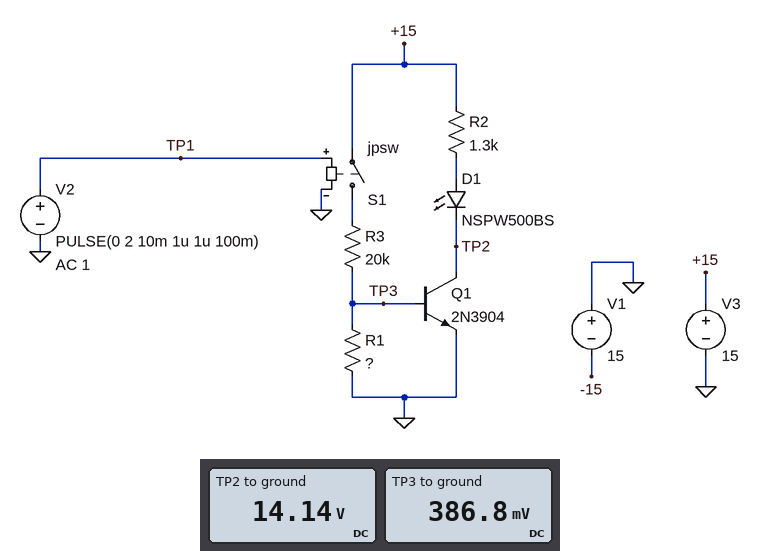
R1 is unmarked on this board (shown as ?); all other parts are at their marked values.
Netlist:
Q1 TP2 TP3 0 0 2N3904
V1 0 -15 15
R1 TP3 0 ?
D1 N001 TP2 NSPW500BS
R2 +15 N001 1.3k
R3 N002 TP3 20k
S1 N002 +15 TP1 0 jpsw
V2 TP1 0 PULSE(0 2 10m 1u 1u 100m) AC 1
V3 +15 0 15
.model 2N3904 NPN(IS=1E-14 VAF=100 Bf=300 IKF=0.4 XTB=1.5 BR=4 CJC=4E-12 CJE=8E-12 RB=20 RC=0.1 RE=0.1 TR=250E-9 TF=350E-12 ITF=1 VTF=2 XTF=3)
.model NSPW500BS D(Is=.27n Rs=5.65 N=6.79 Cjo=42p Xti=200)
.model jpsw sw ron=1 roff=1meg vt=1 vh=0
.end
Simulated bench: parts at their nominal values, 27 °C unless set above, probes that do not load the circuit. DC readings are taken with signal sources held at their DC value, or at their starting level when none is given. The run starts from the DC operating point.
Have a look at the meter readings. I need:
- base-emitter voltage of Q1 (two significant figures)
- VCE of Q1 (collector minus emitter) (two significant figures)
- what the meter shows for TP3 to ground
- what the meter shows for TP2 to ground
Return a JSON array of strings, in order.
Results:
["390 mV", "14 V", "386.8 mV", "14.14 V"]
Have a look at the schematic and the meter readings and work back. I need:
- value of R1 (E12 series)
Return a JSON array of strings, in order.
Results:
["27 kΩ"]
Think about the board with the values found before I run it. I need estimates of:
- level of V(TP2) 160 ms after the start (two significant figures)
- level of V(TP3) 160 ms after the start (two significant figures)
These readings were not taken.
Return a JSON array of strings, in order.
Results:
["14 V", "390 mV"]
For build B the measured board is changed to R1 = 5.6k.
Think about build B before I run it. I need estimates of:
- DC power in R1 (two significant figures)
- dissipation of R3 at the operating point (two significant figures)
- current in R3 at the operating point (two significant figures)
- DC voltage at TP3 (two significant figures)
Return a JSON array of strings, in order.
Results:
["1.2 µW", "4.3 µW", "15 µA", "82 mV"]
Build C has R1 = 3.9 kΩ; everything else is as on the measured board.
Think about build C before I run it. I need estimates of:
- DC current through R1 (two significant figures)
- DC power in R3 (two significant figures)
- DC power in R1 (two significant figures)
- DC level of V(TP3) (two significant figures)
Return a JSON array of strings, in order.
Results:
["15 µA", "4.3 µW", "840 nW", "57 mV"]
